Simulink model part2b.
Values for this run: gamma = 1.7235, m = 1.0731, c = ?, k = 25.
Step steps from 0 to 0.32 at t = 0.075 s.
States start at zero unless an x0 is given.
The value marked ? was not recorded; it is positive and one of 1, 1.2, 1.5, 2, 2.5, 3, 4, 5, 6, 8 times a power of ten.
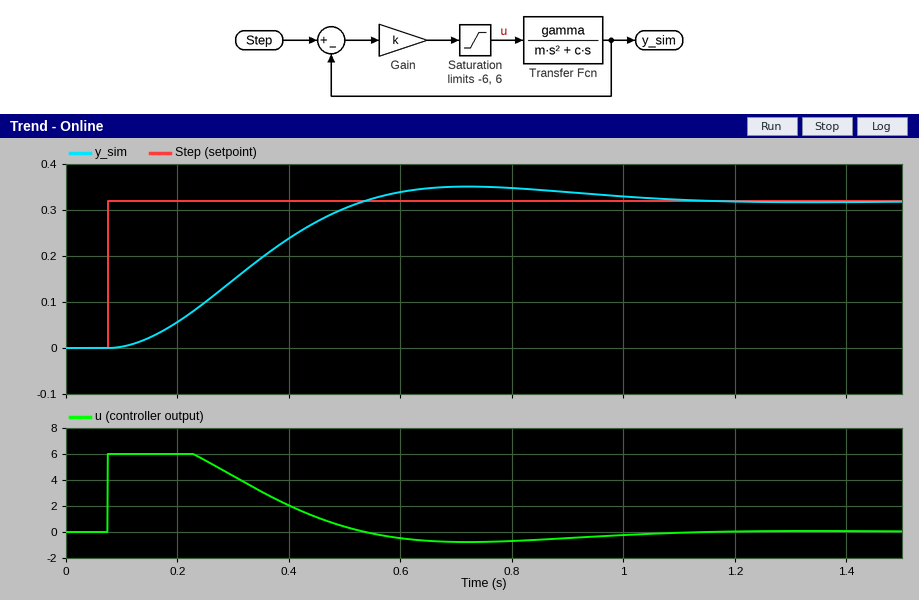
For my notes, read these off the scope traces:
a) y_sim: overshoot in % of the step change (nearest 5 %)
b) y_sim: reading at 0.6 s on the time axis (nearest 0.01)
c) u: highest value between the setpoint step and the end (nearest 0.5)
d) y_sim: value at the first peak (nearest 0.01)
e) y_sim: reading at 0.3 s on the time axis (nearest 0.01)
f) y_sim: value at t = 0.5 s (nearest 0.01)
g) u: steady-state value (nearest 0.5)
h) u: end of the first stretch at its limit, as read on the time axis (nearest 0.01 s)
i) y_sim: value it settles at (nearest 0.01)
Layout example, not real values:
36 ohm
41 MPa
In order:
10 %
0.34
6.0
0.35
0.15
0.30
0.0
0.23 s
0.32
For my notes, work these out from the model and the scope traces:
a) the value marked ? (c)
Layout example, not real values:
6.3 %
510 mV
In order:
8
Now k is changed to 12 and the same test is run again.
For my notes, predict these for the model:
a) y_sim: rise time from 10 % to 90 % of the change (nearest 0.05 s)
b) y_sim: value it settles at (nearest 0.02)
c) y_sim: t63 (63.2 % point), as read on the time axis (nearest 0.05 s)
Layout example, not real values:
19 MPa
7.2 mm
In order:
0.60 s
0.32
0.50 s
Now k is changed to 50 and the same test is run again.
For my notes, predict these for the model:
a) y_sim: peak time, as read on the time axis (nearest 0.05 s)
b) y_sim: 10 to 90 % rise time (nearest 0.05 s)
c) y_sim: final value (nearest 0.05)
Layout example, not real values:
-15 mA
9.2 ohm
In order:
0.60 s
0.25 s
0.30
